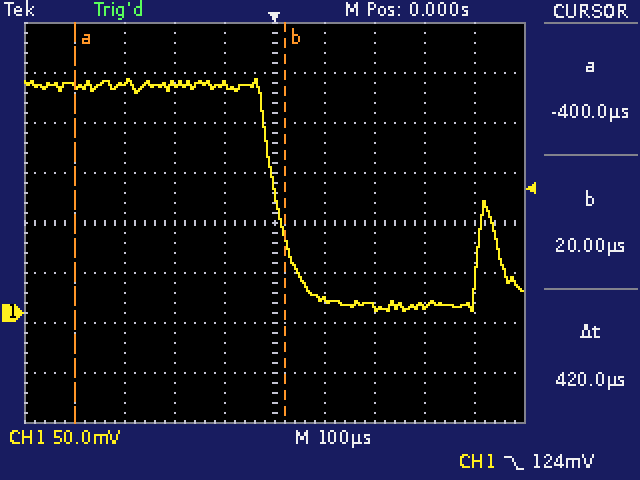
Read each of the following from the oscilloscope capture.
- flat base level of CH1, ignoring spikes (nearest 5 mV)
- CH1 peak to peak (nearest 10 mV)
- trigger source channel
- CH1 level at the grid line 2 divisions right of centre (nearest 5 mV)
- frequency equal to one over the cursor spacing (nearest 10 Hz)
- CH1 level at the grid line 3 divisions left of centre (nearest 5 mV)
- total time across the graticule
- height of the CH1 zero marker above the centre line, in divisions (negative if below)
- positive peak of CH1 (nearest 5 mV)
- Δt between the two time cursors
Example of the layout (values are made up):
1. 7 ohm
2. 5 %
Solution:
1. 10 mV
2. 230 mV
3. CH1
4. 5 mV
5. 2.38 kHz
6. 230 mV
7. 1 ms
8. -1.8 div
9. 235 mV
10. 420 µs
